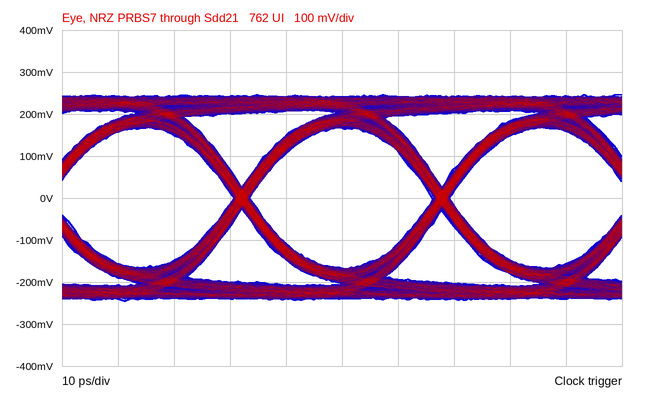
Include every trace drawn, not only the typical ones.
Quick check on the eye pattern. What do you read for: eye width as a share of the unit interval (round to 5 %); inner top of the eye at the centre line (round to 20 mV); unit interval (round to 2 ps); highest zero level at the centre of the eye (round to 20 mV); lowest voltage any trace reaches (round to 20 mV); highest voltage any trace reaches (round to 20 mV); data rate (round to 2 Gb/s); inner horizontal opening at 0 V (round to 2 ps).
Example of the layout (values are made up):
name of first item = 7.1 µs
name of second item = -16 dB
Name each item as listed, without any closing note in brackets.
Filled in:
eye width as a share of the unit interval = 90 %
inner top of the eye at the centre line = 160 mV
unit interval = 36 ps
highest zero level at the centre of the eye = -160 mV
lowest voltage any trace reaches = -240 mV
highest voltage any trace reaches = 240 mV
data rate = 28 Gb/s
inner horizontal opening at 0 V = 32 ps
